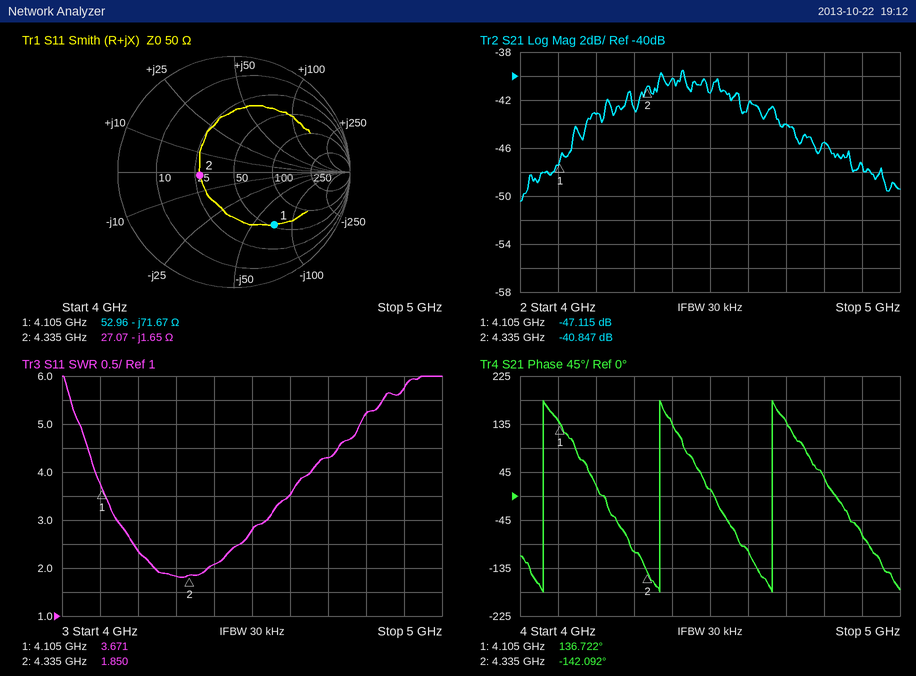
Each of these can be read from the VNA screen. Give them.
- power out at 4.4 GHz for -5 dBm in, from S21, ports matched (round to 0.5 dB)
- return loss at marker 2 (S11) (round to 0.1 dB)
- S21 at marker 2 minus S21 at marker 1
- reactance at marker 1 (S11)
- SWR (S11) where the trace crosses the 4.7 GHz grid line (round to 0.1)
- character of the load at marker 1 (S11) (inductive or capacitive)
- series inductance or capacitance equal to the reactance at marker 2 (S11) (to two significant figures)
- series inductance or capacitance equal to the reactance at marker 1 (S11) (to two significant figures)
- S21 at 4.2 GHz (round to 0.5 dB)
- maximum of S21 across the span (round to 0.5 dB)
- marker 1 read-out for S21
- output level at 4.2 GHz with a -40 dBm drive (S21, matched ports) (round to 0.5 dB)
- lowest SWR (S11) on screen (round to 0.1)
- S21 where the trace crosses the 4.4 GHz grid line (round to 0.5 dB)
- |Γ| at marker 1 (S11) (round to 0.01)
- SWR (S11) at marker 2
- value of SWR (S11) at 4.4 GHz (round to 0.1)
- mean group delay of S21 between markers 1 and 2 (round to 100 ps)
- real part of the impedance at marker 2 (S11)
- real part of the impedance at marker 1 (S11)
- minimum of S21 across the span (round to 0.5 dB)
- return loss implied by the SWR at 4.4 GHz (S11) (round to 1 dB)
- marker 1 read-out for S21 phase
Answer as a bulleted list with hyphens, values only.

- -45.0 dBm
- 10.5 dB
- 6.268 dB
- -71.67 Ω
- 4.3
- capacitive
- 22 pF
- 540 fF
- -43.0 dB
- -39.5 dB
- -47.115 dB
- -83.0 dBm
- 1.8
- -40.0 dB
- 0.57
- 1.850
- 2.1
- 3.4 ns
- 27.07 Ω
- 52.96 Ω
- -50.5 dB
- 9 dB
- 136.722°
